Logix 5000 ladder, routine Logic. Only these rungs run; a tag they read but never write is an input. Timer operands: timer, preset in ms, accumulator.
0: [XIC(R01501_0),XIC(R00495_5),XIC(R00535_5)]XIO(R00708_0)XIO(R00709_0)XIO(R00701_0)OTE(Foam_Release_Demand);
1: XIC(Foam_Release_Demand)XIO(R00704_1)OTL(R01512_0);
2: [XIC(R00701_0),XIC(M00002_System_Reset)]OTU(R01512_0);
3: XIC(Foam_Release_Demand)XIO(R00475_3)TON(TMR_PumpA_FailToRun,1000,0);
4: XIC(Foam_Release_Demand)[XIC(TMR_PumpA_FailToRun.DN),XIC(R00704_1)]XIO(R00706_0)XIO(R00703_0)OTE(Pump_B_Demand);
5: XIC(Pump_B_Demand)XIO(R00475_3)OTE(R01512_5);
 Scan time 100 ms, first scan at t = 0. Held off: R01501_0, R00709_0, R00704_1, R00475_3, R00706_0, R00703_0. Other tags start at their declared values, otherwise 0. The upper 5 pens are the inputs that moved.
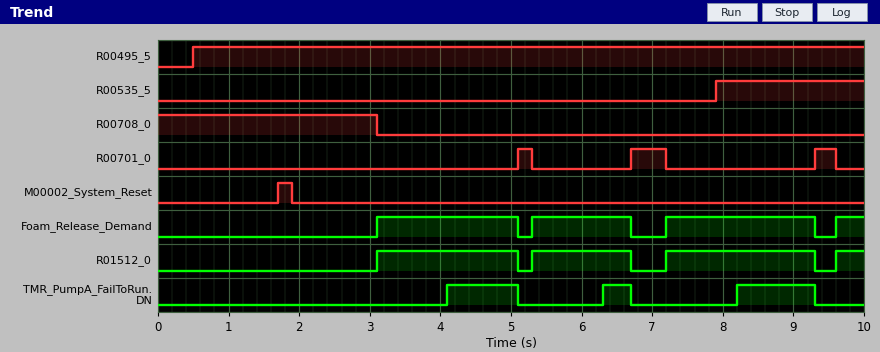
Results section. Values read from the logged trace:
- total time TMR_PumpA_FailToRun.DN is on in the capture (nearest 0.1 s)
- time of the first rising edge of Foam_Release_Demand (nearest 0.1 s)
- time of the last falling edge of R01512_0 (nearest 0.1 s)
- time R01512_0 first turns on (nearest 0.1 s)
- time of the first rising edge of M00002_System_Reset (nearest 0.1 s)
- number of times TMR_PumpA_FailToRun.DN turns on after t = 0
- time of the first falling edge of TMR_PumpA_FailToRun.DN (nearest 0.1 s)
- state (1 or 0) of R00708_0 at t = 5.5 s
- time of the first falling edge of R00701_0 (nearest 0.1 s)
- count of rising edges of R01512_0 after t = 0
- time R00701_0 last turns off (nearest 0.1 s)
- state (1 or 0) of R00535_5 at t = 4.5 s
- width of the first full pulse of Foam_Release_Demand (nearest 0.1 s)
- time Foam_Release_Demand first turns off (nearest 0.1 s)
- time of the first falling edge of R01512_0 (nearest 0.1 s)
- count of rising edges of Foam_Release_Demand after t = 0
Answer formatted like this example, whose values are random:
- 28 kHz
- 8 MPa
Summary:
- 2.5 s
- 3.1 s
- 9.3 s
- 3.1 s
- 1.7 s
- 3
- 5.1 s
- 0
- 5.3 s
- 4
- 9.6 s
- 0
- 2.0 s
- 5.1 s
- 5.1 s
- 4
